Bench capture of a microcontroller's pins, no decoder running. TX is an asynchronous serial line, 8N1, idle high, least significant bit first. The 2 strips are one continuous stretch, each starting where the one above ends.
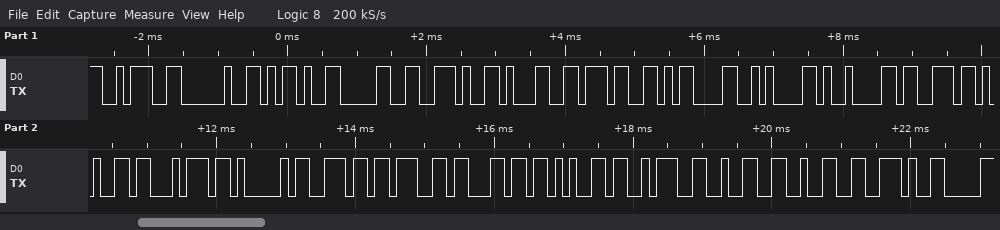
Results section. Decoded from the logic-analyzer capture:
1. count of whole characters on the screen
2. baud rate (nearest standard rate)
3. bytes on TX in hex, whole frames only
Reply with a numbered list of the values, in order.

1. 22
2. 9600 baud
3. 3A 20 2D 30 2E 31 37 0D 0A 09 73 65 74 41 6E 67 6C 65 3A 32 32 2E
